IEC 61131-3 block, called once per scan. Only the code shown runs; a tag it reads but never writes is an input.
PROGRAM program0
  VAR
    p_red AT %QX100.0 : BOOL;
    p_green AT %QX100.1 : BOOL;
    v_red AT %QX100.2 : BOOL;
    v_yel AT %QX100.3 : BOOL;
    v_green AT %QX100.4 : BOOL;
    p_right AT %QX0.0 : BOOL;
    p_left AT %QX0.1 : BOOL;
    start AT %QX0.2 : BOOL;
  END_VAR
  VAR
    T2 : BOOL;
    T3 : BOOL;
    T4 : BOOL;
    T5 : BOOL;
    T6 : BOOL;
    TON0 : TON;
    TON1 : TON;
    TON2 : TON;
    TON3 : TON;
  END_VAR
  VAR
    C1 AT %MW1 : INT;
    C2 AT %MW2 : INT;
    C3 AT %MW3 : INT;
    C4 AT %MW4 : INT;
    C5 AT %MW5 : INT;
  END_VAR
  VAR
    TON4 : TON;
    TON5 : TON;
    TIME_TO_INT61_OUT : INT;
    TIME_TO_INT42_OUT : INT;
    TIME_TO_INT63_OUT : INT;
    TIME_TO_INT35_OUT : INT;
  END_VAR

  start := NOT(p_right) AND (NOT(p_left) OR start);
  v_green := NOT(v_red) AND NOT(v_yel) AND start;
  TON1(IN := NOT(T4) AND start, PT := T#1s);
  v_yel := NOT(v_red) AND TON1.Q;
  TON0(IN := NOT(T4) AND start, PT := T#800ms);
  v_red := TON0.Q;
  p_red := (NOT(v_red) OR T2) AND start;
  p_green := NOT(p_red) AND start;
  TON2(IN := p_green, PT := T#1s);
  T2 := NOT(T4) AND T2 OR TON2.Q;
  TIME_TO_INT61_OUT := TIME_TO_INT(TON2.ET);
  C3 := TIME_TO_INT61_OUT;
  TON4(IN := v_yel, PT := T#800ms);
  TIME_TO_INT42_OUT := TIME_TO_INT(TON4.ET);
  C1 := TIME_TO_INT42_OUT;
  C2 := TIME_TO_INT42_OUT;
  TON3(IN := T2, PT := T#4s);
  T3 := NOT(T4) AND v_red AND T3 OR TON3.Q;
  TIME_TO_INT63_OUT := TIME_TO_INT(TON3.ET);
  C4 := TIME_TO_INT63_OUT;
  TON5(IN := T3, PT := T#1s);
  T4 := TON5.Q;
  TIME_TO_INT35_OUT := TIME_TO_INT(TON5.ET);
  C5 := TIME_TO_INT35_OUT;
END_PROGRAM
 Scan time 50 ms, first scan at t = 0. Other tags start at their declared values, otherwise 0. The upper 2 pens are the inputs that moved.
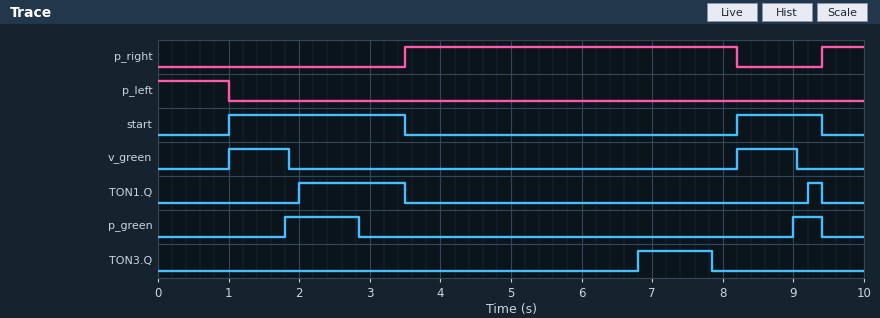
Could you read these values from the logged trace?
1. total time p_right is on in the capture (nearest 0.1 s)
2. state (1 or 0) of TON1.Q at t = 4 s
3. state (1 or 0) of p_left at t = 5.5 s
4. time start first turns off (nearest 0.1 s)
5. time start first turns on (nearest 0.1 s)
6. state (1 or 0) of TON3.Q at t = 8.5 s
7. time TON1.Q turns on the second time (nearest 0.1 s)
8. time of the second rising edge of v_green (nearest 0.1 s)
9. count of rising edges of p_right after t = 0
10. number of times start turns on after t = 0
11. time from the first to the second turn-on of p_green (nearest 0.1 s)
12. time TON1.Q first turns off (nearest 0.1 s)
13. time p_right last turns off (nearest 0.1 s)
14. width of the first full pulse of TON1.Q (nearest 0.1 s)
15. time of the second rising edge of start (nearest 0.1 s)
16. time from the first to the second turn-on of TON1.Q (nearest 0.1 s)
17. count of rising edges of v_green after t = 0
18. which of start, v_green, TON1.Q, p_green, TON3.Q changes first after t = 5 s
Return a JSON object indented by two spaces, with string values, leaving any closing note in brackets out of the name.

{
  "total time p_right is on in the capture": "5.3 s",
  "state (1 or 0) of TON1.Q at t = 4 s": "0",
  "state (1 or 0) of p_left at t = 5.5 s": "0",
  "time start first turns off": "3.5 s",
  "time start first turns on": "1.0 s",
  "state (1 or 0) of TON3.Q at t = 8.5 s": "0",
  "time TON1.Q turns on the second time": "9.2 s",
  "time of the second rising edge of v_green": "8.2 s",
  "count of rising edges of p_right after t = 0": "2",
  "number of times start turns on after t = 0": "2",
  "time from the first to the second turn-on of p_green": "7.2 s",
  "time TON1.Q first turns off": "3.5 s",
  "time p_right last turns off": "8.2 s",
  "width of the first full pulse of TON1.Q": "1.5 s",
  "time of the second rising edge of start": "8.2 s",
  "time from the first to the second turn-on of TON1.Q": "7.2 s",
  "count of rising edges of v_green after t = 0": "2",
  "which of start, v_green, TON1.Q, p_green, TON3.Q changes first after t = 5 s": "TON3.Q"
}
